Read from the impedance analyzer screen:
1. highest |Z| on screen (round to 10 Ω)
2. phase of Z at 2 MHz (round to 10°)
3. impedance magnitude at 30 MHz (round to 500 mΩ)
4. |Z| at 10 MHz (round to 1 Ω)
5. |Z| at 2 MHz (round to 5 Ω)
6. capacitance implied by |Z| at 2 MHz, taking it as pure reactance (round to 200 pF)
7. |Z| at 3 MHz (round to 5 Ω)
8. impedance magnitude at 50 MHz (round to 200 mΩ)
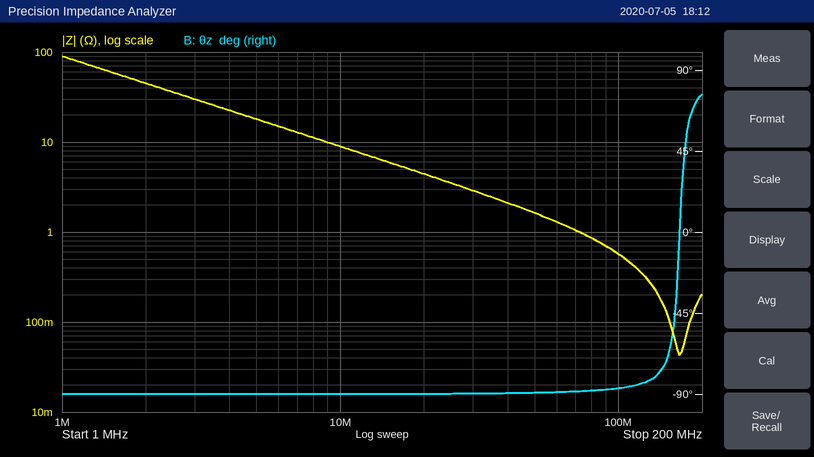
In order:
90 Ω
-90°
3.0 Ω
9 Ω
45 Ω
1.8 nF
30 Ω
1.6 Ω
